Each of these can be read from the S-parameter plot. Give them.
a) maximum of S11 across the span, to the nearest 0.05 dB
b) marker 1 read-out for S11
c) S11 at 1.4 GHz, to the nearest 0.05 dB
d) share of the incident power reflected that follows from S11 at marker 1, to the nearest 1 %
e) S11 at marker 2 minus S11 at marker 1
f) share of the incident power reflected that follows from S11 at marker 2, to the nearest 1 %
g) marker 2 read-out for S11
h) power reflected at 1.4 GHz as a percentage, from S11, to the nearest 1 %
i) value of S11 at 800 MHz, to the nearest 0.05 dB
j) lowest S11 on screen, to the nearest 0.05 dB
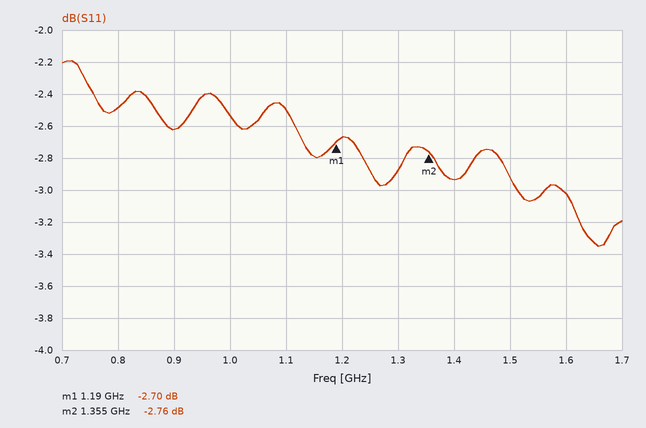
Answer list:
-2.20 dB
-2.70 dB
-2.95 dB
54 %
-0.06 dB
53 %
-2.76 dB
51 %
-2.50 dB
-3.35 dB
